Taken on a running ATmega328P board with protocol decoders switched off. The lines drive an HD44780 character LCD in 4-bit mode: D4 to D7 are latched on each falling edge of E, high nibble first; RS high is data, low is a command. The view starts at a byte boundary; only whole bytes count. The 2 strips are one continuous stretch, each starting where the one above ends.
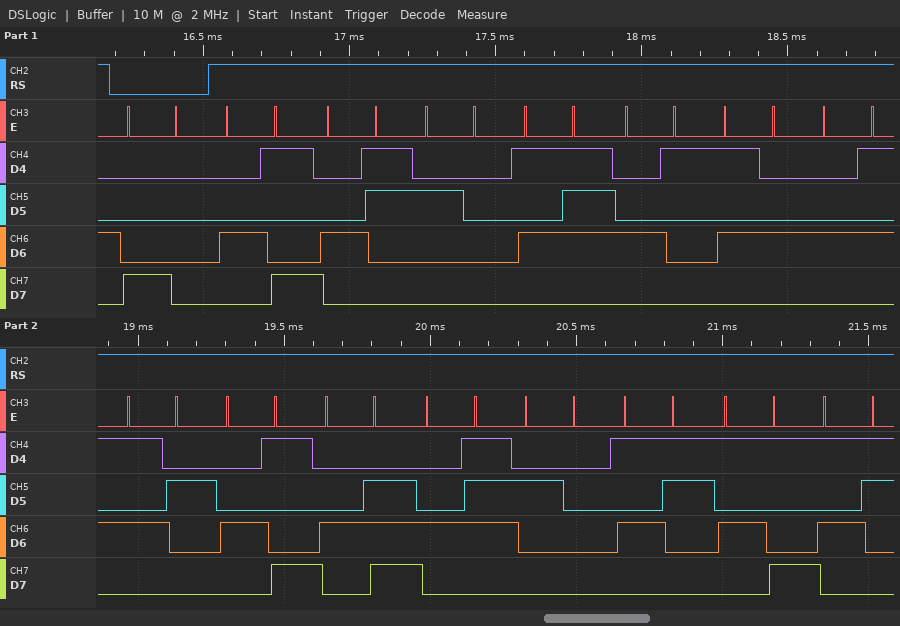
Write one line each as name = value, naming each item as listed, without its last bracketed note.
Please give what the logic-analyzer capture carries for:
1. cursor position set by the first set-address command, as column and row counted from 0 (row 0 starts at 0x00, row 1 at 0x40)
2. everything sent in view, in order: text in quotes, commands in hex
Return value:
cursor position set by the first set-address command, as column and row counted from 0 = column 0, row 0
everything sent in view, in order: text in quotes, commands in hex = 0x80 "IC WATERING SYS"
